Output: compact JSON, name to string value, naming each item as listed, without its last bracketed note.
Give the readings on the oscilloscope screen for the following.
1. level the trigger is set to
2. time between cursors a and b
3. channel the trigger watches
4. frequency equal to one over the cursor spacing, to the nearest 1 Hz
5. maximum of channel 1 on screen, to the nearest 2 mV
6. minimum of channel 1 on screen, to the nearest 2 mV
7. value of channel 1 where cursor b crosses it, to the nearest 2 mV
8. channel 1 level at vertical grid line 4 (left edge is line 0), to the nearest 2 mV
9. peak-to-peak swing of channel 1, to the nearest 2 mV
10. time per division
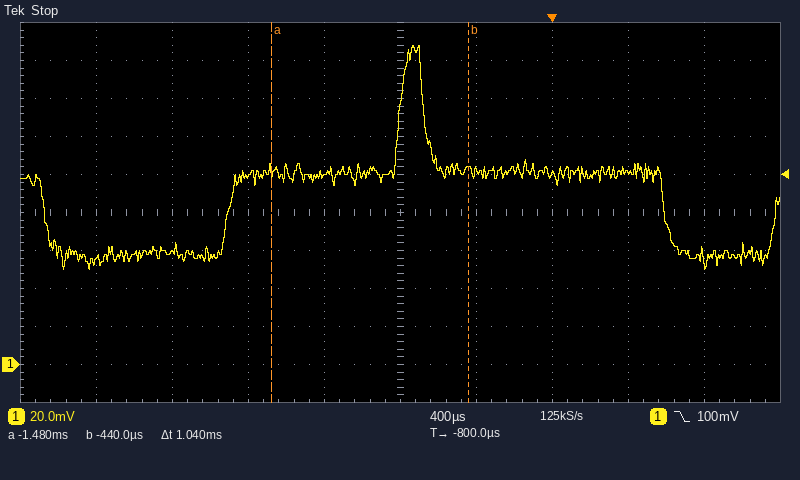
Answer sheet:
{"level the trigger is set to": "100 mV", "time between cursors a and b": "1.04 ms", "channel the trigger watches": "channel 1", "frequency equal to one over the cursor spacing, to the nearest 1 Hz": "962 Hz", "maximum of channel 1 on screen, to the nearest 2 mV": "168 mV", "minimum of channel 1 on screen, to the nearest 2 mV": "50 mV", "value of channel 1 where cursor b crosses it, to the nearest 2 mV": "102 mV", "channel 1 level at vertical grid line 4 (left edge is line 0), to the nearest 2 mV": "100 mV", "peak-to-peak swing of channel 1, to the nearest 2 mV": "118 mV", "time per division": "400 µs"}
